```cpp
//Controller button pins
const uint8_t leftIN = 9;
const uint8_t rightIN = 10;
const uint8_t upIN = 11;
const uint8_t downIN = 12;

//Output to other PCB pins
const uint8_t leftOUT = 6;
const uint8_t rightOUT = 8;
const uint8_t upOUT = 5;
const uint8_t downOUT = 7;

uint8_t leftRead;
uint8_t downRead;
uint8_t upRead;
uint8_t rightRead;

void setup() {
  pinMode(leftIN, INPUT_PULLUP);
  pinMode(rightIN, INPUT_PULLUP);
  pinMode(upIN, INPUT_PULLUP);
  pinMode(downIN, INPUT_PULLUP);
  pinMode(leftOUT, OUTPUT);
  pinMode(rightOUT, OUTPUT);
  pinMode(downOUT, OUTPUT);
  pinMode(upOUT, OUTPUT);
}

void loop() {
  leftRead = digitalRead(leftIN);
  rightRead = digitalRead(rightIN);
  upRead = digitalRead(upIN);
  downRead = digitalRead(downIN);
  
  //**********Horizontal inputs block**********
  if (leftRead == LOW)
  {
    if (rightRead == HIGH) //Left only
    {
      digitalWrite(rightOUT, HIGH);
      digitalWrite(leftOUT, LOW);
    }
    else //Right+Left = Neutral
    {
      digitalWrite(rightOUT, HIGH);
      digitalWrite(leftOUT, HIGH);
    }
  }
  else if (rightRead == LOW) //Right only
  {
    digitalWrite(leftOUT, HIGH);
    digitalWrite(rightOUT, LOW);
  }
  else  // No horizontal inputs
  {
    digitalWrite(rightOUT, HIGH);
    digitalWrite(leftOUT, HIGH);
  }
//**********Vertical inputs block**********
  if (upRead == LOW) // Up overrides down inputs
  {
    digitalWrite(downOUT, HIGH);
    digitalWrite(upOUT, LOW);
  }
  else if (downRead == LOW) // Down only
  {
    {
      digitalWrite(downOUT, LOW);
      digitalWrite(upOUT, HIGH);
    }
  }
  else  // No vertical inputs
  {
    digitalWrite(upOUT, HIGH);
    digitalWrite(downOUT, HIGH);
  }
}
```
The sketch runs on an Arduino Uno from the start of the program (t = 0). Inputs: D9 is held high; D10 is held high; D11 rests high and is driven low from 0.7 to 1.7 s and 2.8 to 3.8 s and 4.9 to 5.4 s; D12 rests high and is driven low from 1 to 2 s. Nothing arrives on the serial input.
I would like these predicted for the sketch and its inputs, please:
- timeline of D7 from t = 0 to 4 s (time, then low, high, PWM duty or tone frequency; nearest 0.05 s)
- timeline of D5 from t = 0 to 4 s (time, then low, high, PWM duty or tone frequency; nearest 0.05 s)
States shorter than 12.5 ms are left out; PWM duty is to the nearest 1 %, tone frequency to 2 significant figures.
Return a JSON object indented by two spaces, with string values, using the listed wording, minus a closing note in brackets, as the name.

{
  "timeline of D7 from t = 0 to 4 s": "0 s high; 1.7 s low; 2 s high",
  "timeline of D5 from t = 0 to 4 s": "0 s high; 0.7 s low; 1.7 s high; 2.8 s low; 3.8 s high"
}
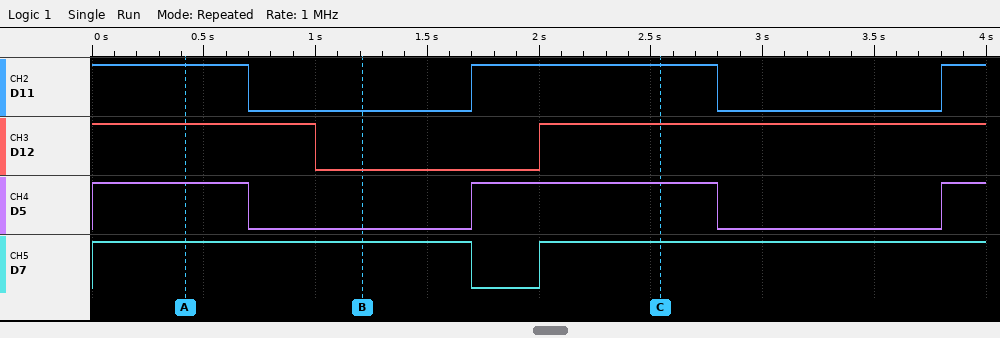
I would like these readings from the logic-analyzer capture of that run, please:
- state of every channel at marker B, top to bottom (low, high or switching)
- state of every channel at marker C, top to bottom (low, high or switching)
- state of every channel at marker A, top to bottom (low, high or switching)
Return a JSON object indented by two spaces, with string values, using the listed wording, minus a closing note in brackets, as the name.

{
  "state of every channel at marker B, top to bottom": "D11 low, D12 low, D5 low, D7 high",
  "state of every channel at marker C, top to bottom": "D11 high, D12 high, D5 high, D7 high",
  "state of every channel at marker A, top to bottom": "D11 high, D12 high, D5 high, D7 high"
}
